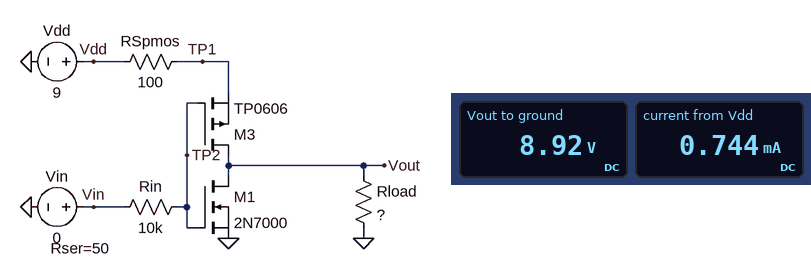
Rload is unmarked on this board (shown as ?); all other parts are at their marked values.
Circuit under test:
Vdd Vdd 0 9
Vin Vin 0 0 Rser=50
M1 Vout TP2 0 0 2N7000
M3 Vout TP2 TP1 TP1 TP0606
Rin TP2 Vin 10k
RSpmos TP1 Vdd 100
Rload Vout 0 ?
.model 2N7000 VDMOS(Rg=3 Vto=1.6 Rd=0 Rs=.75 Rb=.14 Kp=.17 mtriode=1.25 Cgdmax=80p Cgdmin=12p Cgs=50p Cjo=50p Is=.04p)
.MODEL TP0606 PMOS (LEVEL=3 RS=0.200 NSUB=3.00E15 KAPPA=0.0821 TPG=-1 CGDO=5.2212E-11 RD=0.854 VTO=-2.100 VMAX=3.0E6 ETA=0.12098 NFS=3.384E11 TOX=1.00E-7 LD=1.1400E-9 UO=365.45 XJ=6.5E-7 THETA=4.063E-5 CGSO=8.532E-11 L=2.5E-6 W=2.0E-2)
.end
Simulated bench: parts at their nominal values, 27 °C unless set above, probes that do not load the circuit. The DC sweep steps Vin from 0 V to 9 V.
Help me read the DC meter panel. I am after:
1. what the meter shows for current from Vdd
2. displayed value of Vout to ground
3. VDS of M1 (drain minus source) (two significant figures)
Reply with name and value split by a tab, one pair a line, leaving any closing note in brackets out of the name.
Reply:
what the meter shows for current from Vdd	0.744 mA
displayed value of Vout to ground	8.92 V
VDS of M1 (drain minus source)	8.9 V
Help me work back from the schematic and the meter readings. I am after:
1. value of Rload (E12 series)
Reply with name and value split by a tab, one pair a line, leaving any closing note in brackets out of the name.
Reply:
value of Rload	12 kΩ
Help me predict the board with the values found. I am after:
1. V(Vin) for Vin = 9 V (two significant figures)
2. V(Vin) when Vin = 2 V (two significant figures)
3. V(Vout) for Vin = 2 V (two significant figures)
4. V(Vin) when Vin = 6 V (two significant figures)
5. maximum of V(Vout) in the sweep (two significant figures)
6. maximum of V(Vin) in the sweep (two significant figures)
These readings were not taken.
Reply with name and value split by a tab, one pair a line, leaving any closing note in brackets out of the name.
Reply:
V(Vin) for Vin = 9 V	9.0 V
V(Vin) when Vin = 2 V	2.0 V
V(Vout) for Vin = 2 V	7.6 V
V(Vin) when Vin = 6 V	6.0 V
maximum of V(Vout) in the sweep	8.9 V
maximum of V(Vin) in the sweep	9.0 V
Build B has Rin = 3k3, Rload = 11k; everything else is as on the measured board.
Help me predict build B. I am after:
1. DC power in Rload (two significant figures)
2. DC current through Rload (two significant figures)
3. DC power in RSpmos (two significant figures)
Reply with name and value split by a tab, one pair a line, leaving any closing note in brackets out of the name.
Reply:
DC power in Rload	7.2 mW
DC current through Rload	810 µA
DC power in RSpmos	66 µW
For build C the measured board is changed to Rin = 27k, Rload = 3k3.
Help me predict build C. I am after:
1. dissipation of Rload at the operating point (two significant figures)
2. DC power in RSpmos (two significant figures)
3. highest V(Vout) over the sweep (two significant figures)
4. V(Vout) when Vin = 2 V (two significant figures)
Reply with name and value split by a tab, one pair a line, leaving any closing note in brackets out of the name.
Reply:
dissipation of Rload at the operating point	23 mW
DC power in RSpmos	700 µW
highest V(Vout) over the sweep	8.7 V
V(Vout) when Vin = 2 V	7.4 V
